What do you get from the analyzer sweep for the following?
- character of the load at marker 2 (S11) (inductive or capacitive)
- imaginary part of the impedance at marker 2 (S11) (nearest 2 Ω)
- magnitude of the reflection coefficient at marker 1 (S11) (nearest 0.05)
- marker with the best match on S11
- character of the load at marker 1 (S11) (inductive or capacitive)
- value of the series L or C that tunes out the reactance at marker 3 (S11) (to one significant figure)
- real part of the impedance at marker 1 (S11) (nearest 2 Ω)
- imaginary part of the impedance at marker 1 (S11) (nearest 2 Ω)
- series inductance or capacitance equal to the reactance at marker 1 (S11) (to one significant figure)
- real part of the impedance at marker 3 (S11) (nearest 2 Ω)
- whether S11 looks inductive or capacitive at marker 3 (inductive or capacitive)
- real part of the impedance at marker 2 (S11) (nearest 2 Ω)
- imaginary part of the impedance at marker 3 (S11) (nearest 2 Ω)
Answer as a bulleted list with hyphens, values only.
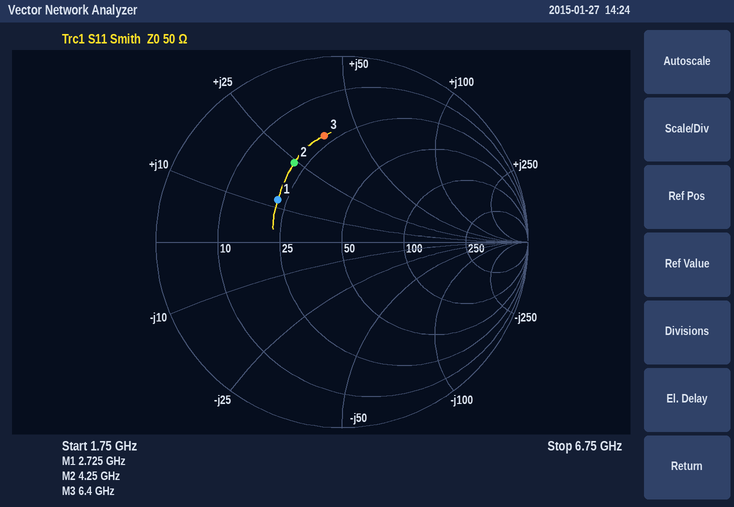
- inductive
- +24 Ω
- 0.40
- marker 1
- inductive
- 700 fF
- 22 Ω
- +12 Ω
- 700 pH
- 22 Ω
- inductive
- 22 Ω
- +38 Ω
